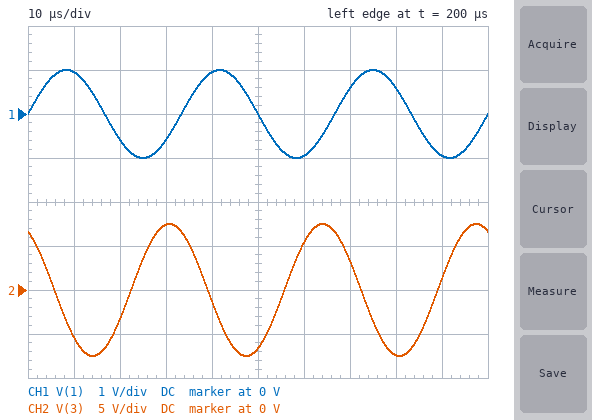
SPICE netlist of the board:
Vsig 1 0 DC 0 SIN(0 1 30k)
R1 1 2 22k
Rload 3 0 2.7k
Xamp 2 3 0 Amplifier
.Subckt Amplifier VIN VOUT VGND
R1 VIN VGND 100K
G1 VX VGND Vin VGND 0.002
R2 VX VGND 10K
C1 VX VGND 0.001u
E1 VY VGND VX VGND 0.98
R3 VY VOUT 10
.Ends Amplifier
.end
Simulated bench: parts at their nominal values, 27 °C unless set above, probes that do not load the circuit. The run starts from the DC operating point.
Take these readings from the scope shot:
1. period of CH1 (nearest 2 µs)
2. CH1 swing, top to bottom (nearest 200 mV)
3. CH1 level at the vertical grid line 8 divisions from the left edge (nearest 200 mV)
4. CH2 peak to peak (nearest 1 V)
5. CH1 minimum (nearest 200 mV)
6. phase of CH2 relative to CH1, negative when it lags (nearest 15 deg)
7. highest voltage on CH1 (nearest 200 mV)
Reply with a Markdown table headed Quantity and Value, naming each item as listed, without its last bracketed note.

| Quantity | Value |
|---|---|
| period of CH1 | 34 µs |
| CH1 swing, top to bottom | 2.0 V |
| CH1 level at the vertical grid line 8 divisions from the left edge | 600 mV |
| CH2 peak to peak | 15 V |
| CH1 minimum | -1.0 V |
| phase of CH2 relative to CH1, negative when it lags | 120 deg |
| highest voltage on CH1 | 1.0 V |
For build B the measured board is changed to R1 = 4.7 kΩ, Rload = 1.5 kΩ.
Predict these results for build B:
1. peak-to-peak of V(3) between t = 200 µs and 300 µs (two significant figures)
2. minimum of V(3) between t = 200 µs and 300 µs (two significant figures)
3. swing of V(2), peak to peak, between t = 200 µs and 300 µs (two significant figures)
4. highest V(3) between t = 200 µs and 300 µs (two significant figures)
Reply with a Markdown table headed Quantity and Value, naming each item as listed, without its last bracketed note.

| Quantity | Value |
|---|---|
| peak-to-peak of V(3) between t = 200 µs and 300 µs | 17 V |
| minimum of V(3) between t = 200 µs and 300 µs | -8.7 V |
| swing of V(2), peak to peak, between t = 200 µs and 300 µs | 1.9 V |
| highest V(3) between t = 200 µs and 300 µs | 8.7 V |
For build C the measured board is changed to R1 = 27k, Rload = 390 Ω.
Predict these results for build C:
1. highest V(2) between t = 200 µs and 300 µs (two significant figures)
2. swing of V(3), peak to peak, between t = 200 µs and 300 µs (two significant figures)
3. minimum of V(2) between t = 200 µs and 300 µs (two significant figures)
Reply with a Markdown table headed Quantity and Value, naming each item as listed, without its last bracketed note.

| Quantity | Value |
|---|---|
| highest V(2) between t = 200 µs and 300 µs | 790 mV |
| swing of V(3), peak to peak, between t = 200 µs and 300 µs | 14 V |
| minimum of V(2) between t = 200 µs and 300 µs | -790 mV |
